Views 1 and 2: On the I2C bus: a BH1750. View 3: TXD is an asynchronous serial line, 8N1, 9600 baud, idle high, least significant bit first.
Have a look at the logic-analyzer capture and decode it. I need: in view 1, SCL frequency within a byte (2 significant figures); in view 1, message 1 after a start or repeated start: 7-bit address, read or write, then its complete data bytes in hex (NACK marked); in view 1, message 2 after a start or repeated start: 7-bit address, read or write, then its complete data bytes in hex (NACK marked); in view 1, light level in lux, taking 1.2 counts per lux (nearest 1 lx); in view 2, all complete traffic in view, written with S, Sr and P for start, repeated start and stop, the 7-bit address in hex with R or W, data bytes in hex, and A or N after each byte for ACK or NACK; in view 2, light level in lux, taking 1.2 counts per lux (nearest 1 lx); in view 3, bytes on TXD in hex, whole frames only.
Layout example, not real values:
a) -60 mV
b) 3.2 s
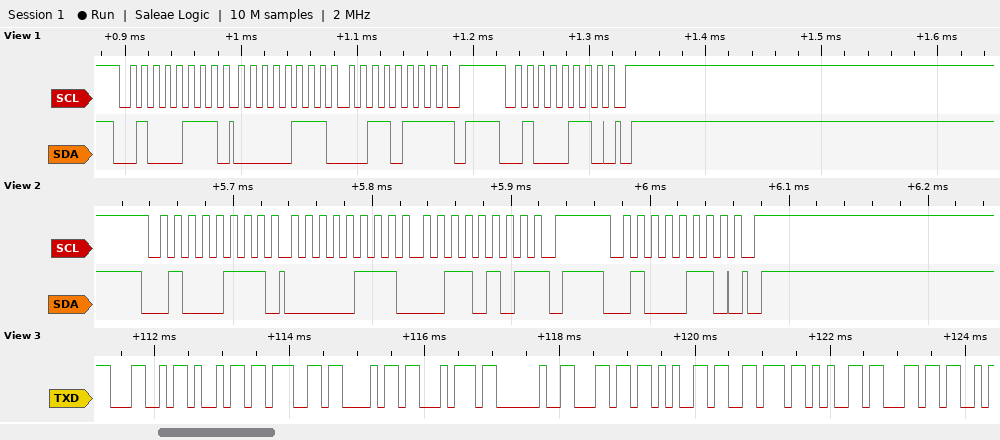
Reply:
a) 100 kHz
b) 0x23 read: 07 37 NACK
c) 0x23 write
d) 1539 lx
e) S 23R A 07 A 35 N P S 23W A P
f) 1538 lx
g) 4C 69 67 68 74 20 6C 65 76 65 6C
